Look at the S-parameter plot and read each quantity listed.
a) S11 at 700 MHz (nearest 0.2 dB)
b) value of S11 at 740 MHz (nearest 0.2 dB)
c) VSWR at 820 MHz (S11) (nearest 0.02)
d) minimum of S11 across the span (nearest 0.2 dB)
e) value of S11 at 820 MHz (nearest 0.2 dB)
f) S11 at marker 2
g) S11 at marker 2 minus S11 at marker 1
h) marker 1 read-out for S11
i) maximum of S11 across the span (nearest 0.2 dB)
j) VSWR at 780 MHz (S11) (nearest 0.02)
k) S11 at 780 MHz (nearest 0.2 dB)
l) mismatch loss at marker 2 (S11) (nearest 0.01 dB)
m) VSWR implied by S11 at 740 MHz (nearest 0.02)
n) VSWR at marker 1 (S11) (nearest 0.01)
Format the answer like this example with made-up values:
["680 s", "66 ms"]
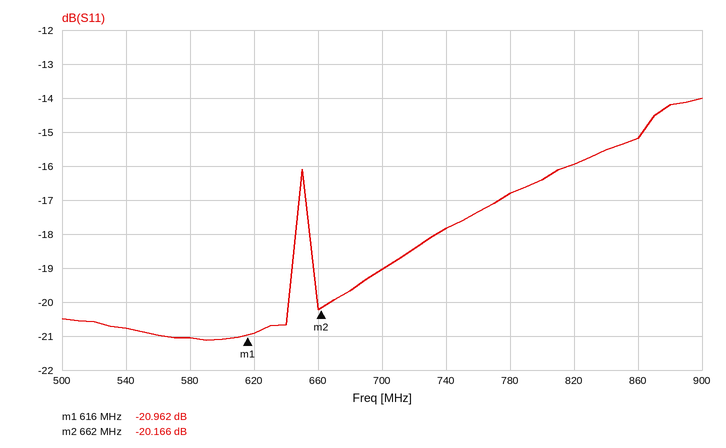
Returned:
["-19.0 dB", "-17.8 dB", "1.38", "-21.2 dB", "-16.0 dB", "-20.166 dB", "0.796 dB", "-20.962 dB", "-14.0 dB", "1.34", "-16.8 dB", "0.04 dB", "1.30", "1.20"]
